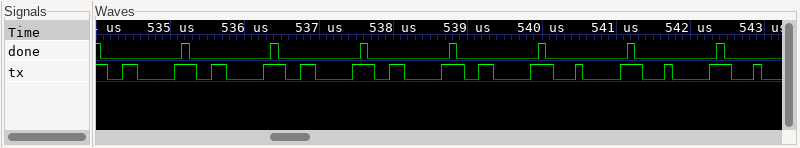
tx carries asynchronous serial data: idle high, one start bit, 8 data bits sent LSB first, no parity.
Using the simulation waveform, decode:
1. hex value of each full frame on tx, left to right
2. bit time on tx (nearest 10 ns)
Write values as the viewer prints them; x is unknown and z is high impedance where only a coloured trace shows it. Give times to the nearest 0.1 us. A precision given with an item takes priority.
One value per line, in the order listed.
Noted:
06, 06, 06, 06, 06, 04, 04
100 ns
